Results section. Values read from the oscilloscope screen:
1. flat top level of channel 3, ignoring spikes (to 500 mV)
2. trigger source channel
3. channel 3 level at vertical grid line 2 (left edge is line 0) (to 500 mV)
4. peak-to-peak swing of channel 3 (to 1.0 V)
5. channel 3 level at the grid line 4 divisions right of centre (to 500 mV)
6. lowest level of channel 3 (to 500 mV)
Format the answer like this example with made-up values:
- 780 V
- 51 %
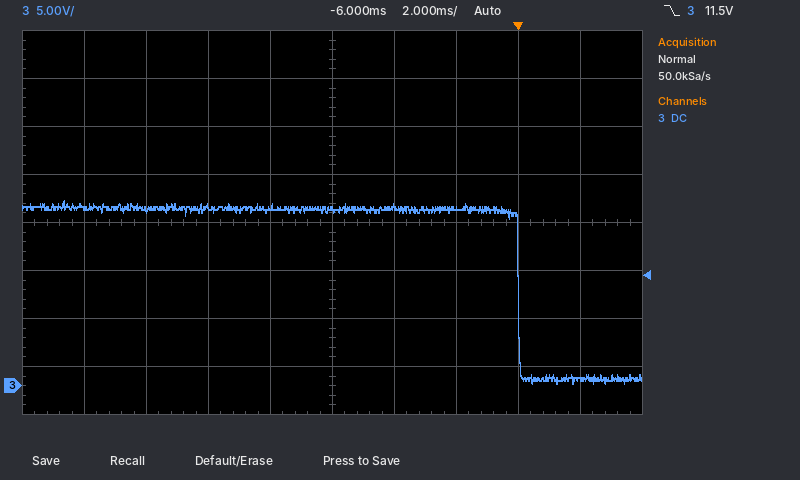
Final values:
- 18.5 V
- channel 3
- 18.5 V
- 19.0 V
- 500 mV
- 0.0 V
